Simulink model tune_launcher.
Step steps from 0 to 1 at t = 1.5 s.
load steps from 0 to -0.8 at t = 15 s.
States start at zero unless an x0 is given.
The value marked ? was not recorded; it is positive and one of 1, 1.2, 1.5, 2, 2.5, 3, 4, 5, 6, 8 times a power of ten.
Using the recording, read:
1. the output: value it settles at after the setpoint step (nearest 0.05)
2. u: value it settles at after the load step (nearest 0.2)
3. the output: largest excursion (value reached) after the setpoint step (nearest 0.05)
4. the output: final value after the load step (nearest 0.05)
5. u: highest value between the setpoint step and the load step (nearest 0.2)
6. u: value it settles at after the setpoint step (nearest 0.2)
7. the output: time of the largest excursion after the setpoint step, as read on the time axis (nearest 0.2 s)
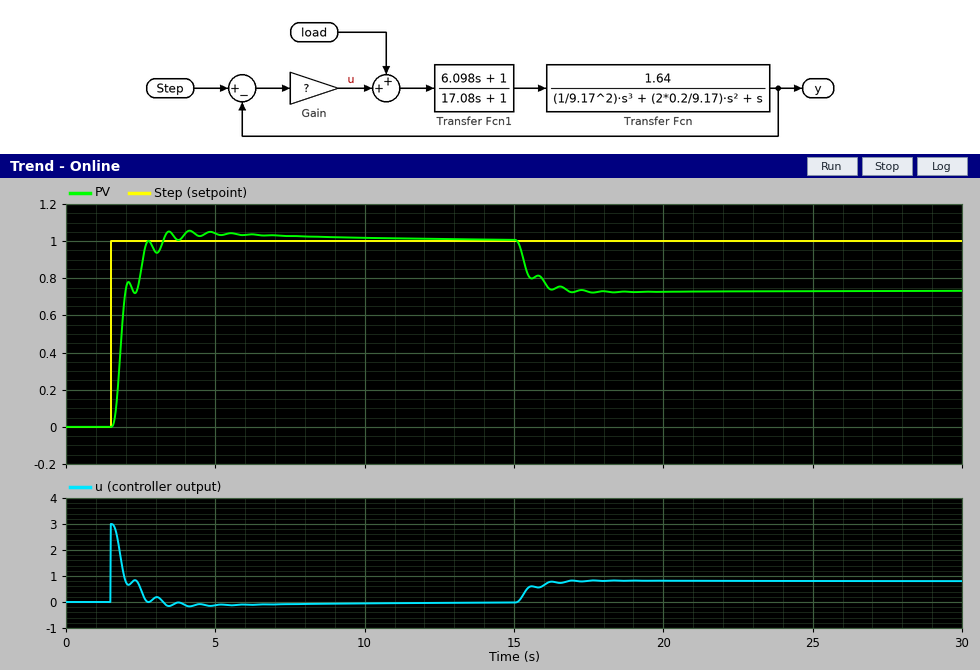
1.00
0.8
1.05
0.75
3.0
0.0
4.2 s
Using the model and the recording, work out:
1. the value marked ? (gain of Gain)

3
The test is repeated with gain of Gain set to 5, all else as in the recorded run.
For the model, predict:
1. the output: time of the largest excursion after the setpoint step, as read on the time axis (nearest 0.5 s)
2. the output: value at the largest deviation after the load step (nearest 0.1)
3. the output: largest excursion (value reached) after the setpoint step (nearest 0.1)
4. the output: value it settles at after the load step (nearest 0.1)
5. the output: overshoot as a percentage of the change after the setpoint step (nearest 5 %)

2.5 s
0.8
1.2
0.8
20 %
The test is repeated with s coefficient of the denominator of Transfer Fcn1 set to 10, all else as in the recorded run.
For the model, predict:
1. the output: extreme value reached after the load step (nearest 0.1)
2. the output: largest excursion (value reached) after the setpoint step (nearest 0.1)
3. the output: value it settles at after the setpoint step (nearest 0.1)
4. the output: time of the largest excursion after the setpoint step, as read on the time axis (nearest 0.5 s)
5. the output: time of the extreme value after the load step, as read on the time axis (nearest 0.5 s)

0.7
1.2
1.0
2.5 s
16.0 s
